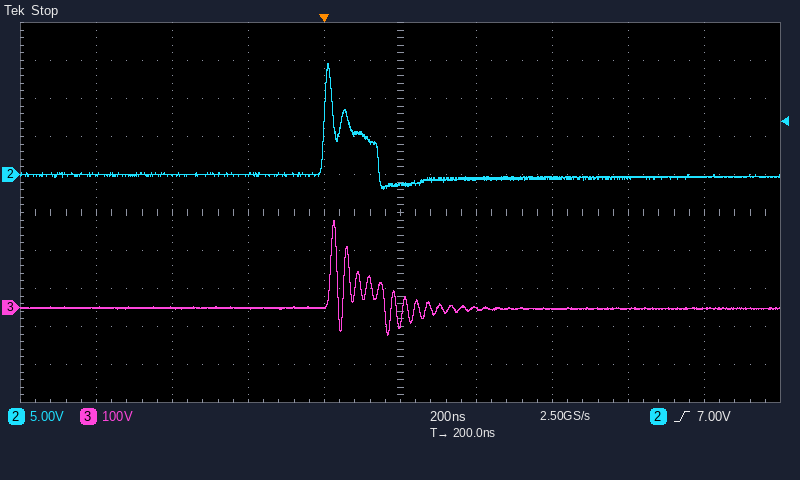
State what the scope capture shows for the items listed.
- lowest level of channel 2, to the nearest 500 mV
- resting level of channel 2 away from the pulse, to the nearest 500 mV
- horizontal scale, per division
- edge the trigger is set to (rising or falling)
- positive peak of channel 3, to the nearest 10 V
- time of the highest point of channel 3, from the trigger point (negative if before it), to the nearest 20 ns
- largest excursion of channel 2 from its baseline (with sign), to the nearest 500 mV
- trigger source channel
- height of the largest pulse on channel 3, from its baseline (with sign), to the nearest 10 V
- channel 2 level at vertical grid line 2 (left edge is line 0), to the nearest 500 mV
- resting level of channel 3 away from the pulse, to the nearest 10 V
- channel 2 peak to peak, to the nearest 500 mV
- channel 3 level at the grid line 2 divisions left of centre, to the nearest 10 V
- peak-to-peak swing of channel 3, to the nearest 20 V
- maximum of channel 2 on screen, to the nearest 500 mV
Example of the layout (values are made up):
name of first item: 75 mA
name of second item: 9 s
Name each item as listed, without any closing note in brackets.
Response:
lowest level of channel 2, to the nearest 500 mV: -2.0 V
resting level of channel 2 away from the pulse, to the nearest 500 mV: -500 mV
horizontal scale, per division: 200 ns
edge the trigger is set to: rising
positive peak of channel 3, to the nearest 10 V: 230 V
time of the highest point of channel 3, from the trigger point (negative if before it), to the nearest 20 ns: +20 ns
largest excursion of channel 2 from its baseline (with sign), to the nearest 500 mV: +15.0 V
trigger source channel: channel 2
height of the largest pulse on channel 3, from its baseline (with sign), to the nearest 10 V: +230 V
channel 2 level at vertical grid line 2 (left edge is line 0), to the nearest 500 mV: 0.0 V
resting level of channel 3 away from the pulse, to the nearest 10 V: 0 V
channel 2 peak to peak, to the nearest 500 mV: 16.5 V
channel 3 level at the grid line 2 divisions left of centre, to the nearest 10 V: 0 V
peak-to-peak swing of channel 3, to the nearest 20 V: 300 V
maximum of channel 2 on screen, to the nearest 500 mV: 14.5 V
